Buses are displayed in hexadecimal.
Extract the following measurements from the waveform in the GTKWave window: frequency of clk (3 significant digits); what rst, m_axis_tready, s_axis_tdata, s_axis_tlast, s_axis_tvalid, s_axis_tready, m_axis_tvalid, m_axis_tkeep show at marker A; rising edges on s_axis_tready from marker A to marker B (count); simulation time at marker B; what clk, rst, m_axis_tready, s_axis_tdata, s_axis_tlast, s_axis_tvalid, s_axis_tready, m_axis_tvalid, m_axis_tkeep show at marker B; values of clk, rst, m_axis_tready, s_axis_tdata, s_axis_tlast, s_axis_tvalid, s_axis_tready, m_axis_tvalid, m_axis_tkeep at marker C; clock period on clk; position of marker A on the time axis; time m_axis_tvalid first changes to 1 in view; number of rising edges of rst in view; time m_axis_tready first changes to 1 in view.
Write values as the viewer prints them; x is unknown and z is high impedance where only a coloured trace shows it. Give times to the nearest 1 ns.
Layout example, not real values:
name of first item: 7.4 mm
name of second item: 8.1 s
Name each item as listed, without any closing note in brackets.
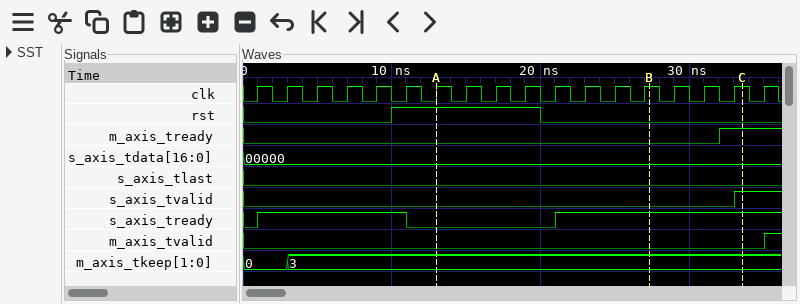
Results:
frequency of clk: 500 MHz
what rst, m_axis_tready, s_axis_tdata, s_axis_tlast, s_axis_tvalid, s_axis_tready, m_axis_tvalid, m_axis_tkeep show at marker A: rst=1, m_axis_tready=0, s_axis_tdata=00000, s_axis_tlast=0, s_axis_tvalid=0, s_axis_tready=0, m_axis_tvalid=0, m_axis_tkeep=3
rising edges on s_axis_tready from marker A to marker B: 1
simulation time at marker B: 27 ns
what clk, rst, m_axis_tready, s_axis_tdata, s_axis_tlast, s_axis_tvalid, s_axis_tready, m_axis_tvalid, m_axis_tkeep show at marker B: clk=1, rst=0, m_axis_tready=0, s_axis_tdata=00000, s_axis_tlast=0, s_axis_tvalid=0, s_axis_tready=1, m_axis_tvalid=0, m_axis_tkeep=3
values of clk, rst, m_axis_tready, s_axis_tdata, s_axis_tlast, s_axis_tvalid, s_axis_tready, m_axis_tvalid, m_axis_tkeep at marker C: clk=1, rst=0, m_axis_tready=1, s_axis_tdata=00000, s_axis_tlast=0, s_axis_tvalid=1, s_axis_tready=1, m_axis_tvalid=0, m_axis_tkeep=3
clock period on clk: 2 ns
position of marker A on the time axis: 13 ns
time m_axis_tvalid first changes to 1 in view: 35 ns
number of rising edges of rst in view: 1
time m_axis_tready first changes to 1 in view: 32 ns
